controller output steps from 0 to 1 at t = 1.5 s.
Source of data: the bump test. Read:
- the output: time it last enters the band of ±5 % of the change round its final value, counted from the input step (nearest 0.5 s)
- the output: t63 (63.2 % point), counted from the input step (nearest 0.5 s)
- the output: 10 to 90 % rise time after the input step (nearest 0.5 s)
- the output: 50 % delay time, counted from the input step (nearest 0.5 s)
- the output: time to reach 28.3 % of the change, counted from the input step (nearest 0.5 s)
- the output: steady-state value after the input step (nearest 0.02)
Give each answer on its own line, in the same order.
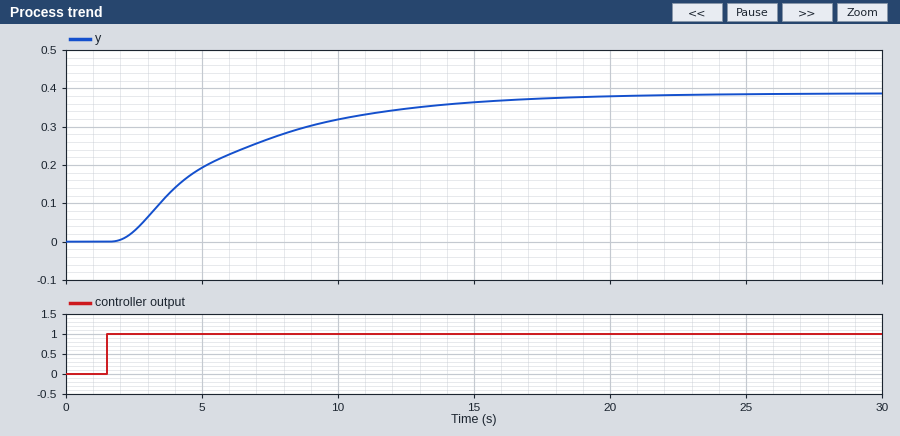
14.5 s
5.0 s
10.0 s
3.5 s
2.0 s
0.38
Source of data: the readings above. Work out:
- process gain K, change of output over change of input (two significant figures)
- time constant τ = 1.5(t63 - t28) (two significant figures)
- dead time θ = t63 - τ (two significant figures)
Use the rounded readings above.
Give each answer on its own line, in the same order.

0.38
4.5 s
0.50 s
